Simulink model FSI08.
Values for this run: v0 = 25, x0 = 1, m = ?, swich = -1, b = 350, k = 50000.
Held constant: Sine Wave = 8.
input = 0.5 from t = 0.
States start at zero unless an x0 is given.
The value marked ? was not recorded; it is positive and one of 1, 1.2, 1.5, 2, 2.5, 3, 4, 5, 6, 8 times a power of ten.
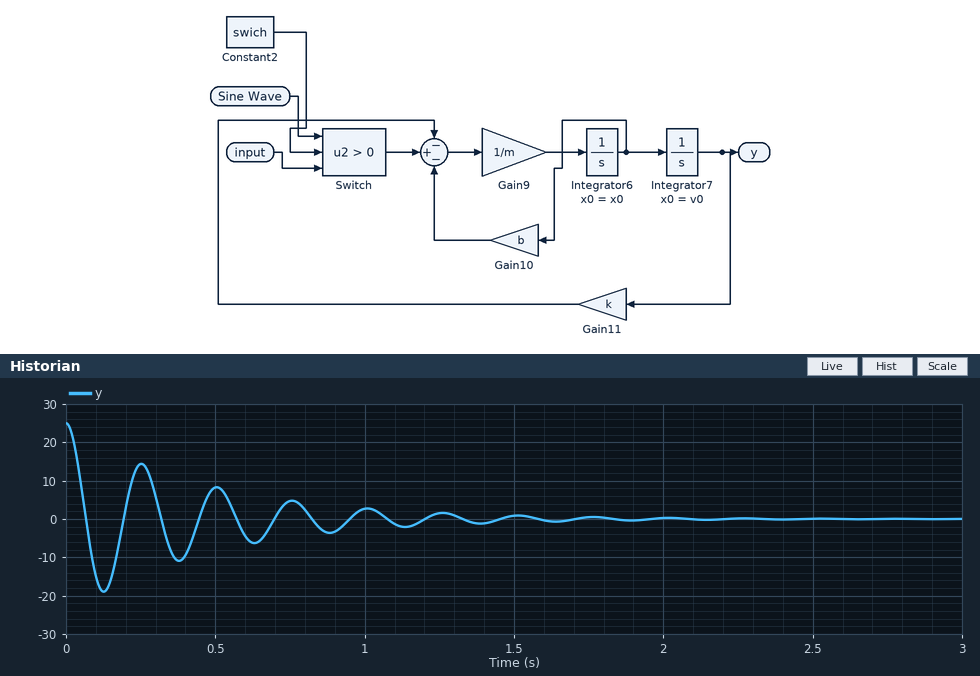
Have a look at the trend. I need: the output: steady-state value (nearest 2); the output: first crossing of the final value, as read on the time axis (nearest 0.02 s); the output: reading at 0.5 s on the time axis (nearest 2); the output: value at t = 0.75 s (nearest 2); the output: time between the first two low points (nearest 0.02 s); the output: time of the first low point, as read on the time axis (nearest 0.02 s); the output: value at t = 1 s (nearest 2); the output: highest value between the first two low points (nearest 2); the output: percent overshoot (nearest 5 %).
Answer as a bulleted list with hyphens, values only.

- 0
- 0.06 s
- 8
- 4
- 0.26 s
- 0.12 s
- 2
- 14
- 75 %
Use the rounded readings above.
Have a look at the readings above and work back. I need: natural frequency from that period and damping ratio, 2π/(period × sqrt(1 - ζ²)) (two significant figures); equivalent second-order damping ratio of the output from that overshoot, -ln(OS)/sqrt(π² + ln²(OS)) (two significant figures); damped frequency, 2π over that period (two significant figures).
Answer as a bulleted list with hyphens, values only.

- 24 rad/s
- 0.091
- 24 rad/s
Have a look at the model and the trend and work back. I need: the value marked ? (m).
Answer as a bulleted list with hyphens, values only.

- 80
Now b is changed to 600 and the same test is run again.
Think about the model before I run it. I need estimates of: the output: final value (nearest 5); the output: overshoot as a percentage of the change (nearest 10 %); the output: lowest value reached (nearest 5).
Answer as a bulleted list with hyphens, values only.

- 0
- 60 %
- -15
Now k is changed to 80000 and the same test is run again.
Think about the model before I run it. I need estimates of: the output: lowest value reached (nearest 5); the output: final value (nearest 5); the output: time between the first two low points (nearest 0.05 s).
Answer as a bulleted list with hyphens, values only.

- -20
- 0
- 0.20 s
